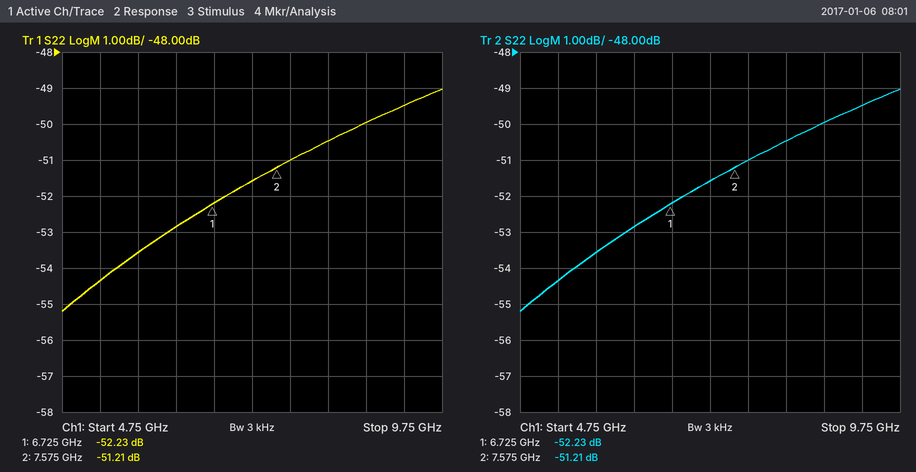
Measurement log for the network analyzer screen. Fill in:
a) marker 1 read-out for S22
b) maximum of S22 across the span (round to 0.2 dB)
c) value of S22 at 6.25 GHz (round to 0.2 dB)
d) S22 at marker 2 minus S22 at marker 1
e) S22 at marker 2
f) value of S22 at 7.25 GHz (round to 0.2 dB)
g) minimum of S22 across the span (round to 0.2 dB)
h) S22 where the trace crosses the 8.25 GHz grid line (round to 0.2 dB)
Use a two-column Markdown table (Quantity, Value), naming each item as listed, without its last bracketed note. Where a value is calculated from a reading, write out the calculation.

| Quantity | Value |
|---|---|
| marker 1 read-out for S22 | -52.23 dB |
| maximum of S22 across the span | -49.0 dB |
| value of S22 at 6.25 GHz | -52.8 dB |
| S22 at marker 2 minus S22 at marker 1 | -51.21 − (-52.23) = 1.02 dB |
| S22 at marker 2 | -51.21 dB |
| value of S22 at 7.25 GHz | -51.6 dB |
| minimum of S22 across the span | -55.2 dB |
| S22 where the trace crosses the 8.25 GHz grid line | -50.4 dB |
